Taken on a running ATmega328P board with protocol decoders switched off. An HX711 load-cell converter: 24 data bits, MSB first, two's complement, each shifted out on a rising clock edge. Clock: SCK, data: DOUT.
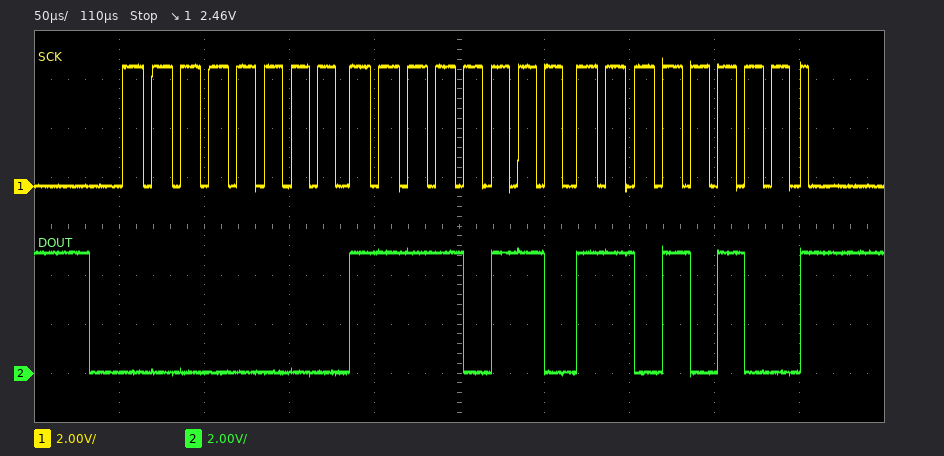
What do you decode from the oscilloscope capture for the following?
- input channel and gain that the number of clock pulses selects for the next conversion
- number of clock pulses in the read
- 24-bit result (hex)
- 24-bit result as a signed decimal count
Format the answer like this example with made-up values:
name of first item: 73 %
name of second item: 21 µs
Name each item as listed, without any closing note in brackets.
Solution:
input channel and gain that the number of clock pulses selects for the next conversion: channel A, gain 128
number of clock pulses in the read: 25
24-bit result: 0x00F6D4
24-bit result as a signed decimal count: 63188
